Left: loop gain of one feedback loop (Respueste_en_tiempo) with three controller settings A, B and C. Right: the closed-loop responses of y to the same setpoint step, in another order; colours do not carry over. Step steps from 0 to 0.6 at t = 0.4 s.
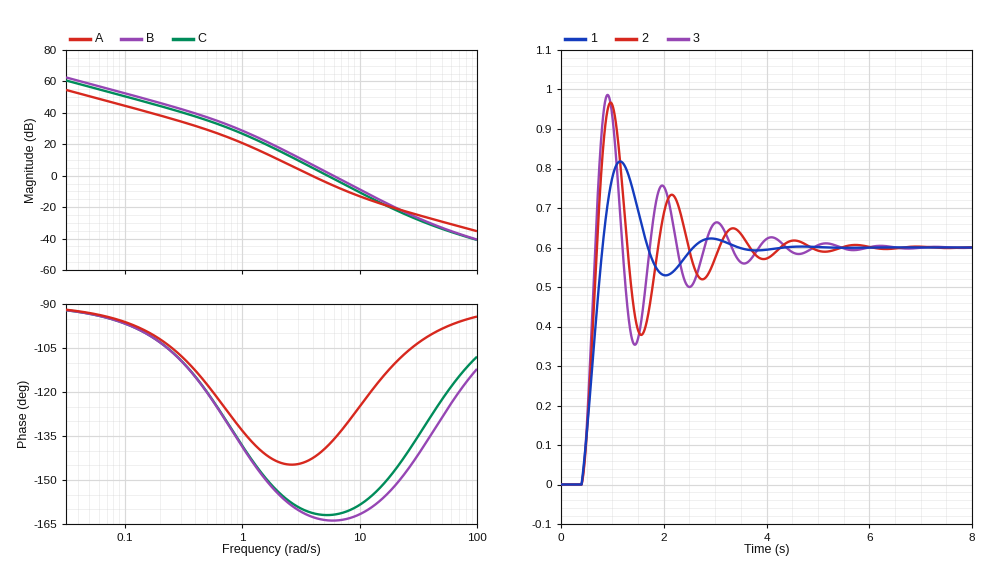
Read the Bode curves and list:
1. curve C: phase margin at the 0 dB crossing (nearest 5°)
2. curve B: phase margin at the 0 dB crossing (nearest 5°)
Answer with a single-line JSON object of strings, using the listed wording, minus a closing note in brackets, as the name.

{"curve C: phase margin at the 0 dB crossing": "20°", "curve B: phase margin at the 0 dB crossing": "15°"}
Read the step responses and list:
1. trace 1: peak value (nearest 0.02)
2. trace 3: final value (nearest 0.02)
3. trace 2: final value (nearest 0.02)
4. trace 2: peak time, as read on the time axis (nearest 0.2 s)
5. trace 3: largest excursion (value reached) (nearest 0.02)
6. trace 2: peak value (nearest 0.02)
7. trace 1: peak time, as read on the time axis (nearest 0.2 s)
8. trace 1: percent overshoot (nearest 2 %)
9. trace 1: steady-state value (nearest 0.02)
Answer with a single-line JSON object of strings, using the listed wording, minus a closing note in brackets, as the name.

{"trace 1: peak value": "0.82", "trace 3: final value": "0.60", "trace 2: final value": "0.60", "trace 2: peak time, as read on the time axis": "1.0 s", "trace 3: largest excursion (value reached)": "0.98", "trace 2: peak value": "0.96", "trace 1: peak time, as read on the time axis": "1.2 s", "trace 1: percent overshoot": "36 %", "trace 1: steady-state value": "0.60"}
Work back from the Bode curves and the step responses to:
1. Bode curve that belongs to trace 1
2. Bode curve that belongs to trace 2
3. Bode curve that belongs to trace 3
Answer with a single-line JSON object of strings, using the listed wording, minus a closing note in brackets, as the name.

{"Bode curve that belongs to trace 1": "A", "Bode curve that belongs to trace 2": "C", "Bode curve that belongs to trace 3": "B"}
